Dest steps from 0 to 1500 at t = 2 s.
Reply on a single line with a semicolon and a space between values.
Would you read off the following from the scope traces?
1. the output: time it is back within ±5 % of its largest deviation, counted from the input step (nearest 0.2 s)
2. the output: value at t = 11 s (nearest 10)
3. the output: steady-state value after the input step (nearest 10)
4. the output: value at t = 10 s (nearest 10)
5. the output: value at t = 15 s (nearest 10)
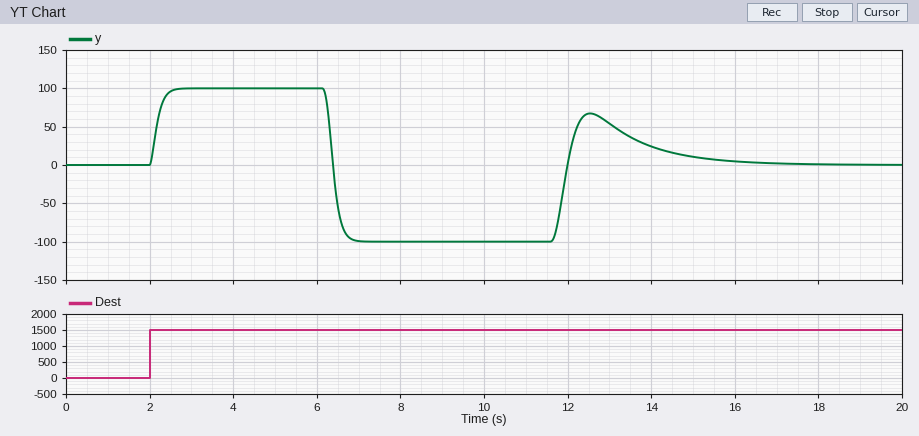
14.0 s; -100; 0; -100; 10
